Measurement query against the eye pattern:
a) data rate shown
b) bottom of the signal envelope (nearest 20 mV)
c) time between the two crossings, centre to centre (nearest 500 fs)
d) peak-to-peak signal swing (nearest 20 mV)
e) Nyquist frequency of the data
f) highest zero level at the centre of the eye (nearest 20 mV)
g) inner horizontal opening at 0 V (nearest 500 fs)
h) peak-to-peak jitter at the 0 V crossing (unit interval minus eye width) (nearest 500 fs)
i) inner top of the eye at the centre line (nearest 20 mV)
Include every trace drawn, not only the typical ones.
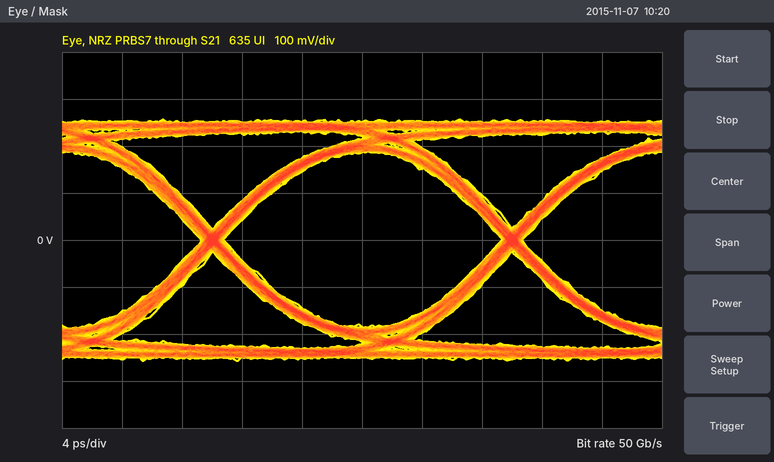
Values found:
50 Gb/s
-260 mV
20.0 ps
520 mV
25 GHz
-180 mV
18.5 ps
1.5 ps
180 mV
